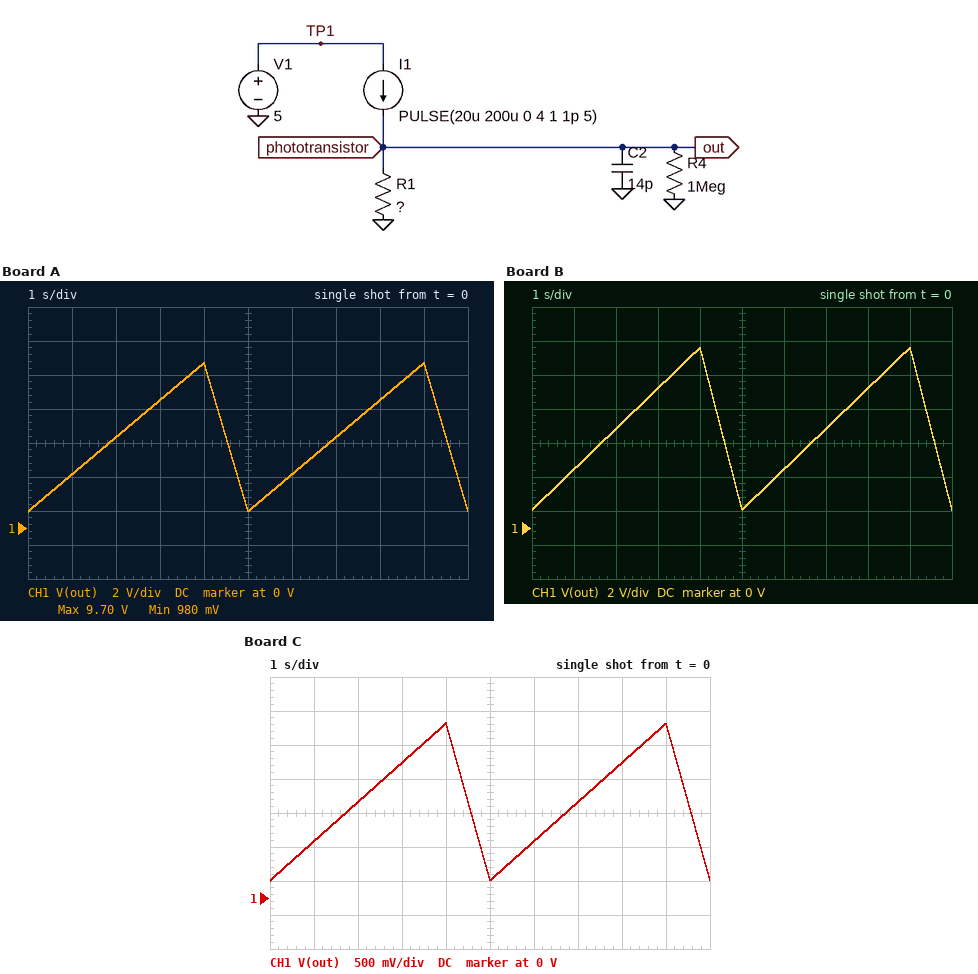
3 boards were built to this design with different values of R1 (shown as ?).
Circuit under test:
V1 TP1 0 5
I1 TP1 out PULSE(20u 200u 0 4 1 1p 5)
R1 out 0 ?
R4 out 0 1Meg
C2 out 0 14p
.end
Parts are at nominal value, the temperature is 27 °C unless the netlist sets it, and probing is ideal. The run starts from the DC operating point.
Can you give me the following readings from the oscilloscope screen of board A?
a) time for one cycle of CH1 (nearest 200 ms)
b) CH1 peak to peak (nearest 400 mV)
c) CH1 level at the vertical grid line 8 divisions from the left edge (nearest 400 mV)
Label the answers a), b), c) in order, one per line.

a) 5.0 s
b) 8.8 V
c) 7.6 V
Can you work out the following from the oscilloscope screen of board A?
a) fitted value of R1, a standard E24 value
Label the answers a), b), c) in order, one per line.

a) 51 kΩ
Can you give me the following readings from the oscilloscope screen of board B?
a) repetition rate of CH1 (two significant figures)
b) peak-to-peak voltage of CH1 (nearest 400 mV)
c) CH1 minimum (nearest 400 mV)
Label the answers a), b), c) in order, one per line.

a) 200 mHz
b) 9.6 V
c) 1.2 V
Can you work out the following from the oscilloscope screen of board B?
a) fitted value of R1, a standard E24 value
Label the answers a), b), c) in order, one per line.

a) 56 kΩ
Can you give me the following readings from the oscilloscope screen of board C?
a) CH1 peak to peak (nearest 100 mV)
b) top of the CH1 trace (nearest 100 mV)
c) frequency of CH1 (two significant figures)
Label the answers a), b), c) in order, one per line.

a) 2.3 V
b) 2.6 V
c) 200 mHz
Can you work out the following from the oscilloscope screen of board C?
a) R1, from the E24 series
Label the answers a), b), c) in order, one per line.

a) 13 kΩ
